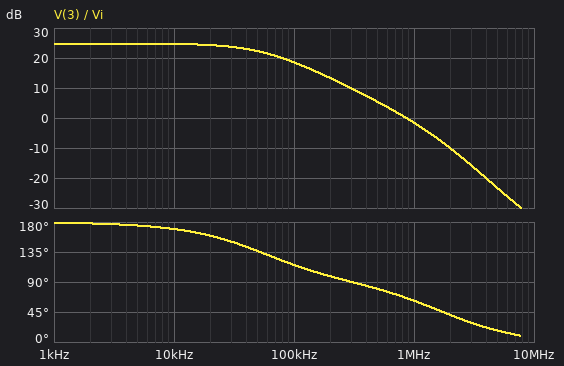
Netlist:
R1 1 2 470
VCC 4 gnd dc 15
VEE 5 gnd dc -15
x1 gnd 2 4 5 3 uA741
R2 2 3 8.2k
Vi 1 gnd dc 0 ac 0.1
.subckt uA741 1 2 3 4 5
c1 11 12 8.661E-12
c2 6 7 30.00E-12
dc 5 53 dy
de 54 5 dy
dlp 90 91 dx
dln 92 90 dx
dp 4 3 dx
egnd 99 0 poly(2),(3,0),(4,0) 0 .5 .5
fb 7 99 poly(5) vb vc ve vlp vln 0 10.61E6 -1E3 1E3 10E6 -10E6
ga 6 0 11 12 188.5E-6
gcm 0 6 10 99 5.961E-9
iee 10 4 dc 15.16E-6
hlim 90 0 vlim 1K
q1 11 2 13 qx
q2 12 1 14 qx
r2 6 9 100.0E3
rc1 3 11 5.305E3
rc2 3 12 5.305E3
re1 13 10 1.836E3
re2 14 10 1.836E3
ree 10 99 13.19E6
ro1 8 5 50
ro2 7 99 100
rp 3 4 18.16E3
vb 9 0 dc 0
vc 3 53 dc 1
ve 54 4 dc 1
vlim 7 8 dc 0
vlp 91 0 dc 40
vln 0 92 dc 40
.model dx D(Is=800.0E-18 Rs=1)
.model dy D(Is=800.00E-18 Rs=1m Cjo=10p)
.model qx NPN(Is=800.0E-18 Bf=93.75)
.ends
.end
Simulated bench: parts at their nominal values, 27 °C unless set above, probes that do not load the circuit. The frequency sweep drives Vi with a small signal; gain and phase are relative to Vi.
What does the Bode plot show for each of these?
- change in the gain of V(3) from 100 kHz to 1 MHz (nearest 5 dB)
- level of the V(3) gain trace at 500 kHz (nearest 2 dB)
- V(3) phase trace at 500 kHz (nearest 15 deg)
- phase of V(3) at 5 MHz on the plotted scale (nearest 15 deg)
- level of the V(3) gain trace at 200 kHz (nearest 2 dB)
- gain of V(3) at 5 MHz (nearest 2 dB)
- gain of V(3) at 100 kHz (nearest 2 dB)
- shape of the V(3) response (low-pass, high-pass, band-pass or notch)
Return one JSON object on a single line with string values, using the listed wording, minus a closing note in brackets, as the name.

{"change in the gain of V(3) from 100 kHz to 1 MHz": "-20 dB", "level of the V(3) gain trace at 500 kHz": "6 dB", "V(3) phase trace at 500 kHz": "75 deg", "phase of V(3) at 5 MHz on the plotted scale": "15 deg", "level of the V(3) gain trace at 200 kHz": "14 dB", "gain of V(3) at 5 MHz": "-24 dB", "gain of V(3) at 100 kHz": "18 dB", "shape of the V(3) response": "low-pass"}
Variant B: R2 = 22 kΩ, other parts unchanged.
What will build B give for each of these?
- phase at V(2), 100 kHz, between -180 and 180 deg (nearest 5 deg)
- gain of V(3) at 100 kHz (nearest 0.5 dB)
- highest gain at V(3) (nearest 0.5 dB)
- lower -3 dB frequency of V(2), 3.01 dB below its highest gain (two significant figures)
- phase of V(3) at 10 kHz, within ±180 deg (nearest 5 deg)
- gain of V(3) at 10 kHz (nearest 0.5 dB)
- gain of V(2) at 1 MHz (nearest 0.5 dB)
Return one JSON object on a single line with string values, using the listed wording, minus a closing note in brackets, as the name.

{"phase at V(2), 100 kHz, between -180 and 180 deg": "10 deg", "gain of V(3) at 100 kHz": "19.5 dB", "highest gain at V(3)": "33.5 dB", "lower -3 dB frequency of V(2), 3.01 dB below its highest gain": "21 kHz", "phase of V(3) at 10 kHz, within ±180 deg": "155 deg", "gain of V(3) at 10 kHz": "32.5 dB", "gain of V(2) at 1 MHz": "0 dB"}
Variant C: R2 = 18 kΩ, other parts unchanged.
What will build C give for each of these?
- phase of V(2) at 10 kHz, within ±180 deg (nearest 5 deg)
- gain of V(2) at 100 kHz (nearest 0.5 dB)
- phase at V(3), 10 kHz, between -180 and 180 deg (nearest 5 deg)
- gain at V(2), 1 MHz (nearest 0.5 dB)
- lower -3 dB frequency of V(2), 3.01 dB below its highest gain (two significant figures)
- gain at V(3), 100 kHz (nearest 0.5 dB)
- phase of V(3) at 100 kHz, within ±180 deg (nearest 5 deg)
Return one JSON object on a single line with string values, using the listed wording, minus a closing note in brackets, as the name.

{"phase of V(2) at 10 kHz, within ±180 deg": "70 deg", "gain of V(2) at 100 kHz": "-0.5 dB", "phase at V(3), 10 kHz, between -180 and 180 deg": "160 deg", "gain at V(2), 1 MHz": "0 dB", "lower -3 dB frequency of V(2), 3.01 dB below its highest gain": "26 kHz", "gain at V(3), 100 kHz": "19.5 dB", "phase of V(3) at 100 kHz, within ±180 deg": "100 deg"}
